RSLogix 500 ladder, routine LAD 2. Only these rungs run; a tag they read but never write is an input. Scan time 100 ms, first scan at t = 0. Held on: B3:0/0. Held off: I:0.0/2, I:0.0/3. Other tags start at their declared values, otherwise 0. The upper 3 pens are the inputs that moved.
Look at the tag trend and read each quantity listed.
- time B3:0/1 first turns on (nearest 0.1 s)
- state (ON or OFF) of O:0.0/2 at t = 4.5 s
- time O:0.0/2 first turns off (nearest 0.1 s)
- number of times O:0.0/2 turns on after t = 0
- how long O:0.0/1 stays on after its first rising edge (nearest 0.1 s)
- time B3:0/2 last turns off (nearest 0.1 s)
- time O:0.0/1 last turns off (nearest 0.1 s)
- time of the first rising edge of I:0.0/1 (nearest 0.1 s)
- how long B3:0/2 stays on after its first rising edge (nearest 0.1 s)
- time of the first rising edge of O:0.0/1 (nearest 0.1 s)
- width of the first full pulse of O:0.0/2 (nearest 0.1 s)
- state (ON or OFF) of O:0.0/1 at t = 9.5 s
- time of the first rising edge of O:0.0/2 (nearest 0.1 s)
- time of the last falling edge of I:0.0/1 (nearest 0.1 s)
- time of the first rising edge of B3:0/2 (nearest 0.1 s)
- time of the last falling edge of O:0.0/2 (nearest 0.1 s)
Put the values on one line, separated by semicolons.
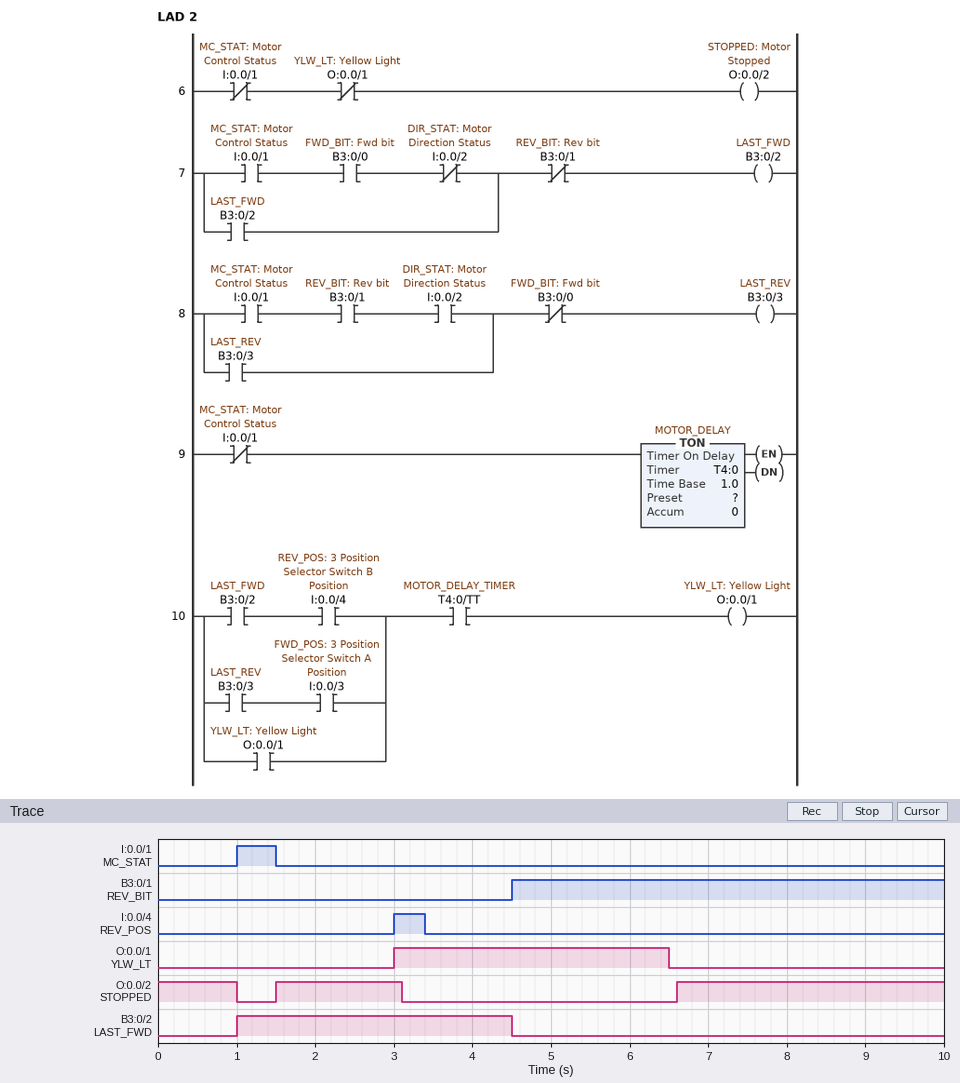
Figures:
4.5 s; OFF; 1.0 s; 2; 3.5 s; 4.5 s; 6.5 s; 1.0 s; 3.5 s; 3.0 s; 1.6 s; OFF; 1.5 s; 1.5 s; 1.0 s; 3.1 s
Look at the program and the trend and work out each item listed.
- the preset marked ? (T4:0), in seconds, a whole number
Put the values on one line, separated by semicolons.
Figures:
5 s
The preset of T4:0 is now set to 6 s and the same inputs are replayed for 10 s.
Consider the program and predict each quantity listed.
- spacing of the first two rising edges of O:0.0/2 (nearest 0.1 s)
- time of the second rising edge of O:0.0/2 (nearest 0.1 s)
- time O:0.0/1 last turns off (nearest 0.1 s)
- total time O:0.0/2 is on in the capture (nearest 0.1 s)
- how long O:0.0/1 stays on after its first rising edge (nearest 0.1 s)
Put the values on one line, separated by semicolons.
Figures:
6.1 s; 7.6 s; 7.5 s; 5.0 s; 4.5 s
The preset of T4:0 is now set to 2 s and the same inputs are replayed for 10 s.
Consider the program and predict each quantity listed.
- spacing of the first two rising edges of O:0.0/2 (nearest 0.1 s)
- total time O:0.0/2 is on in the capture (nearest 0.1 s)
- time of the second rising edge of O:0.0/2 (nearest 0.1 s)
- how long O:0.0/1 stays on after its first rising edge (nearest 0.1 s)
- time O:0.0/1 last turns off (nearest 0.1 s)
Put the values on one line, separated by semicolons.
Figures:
2.1 s; 9.0 s; 3.6 s; 0.5 s; 3.5 s
